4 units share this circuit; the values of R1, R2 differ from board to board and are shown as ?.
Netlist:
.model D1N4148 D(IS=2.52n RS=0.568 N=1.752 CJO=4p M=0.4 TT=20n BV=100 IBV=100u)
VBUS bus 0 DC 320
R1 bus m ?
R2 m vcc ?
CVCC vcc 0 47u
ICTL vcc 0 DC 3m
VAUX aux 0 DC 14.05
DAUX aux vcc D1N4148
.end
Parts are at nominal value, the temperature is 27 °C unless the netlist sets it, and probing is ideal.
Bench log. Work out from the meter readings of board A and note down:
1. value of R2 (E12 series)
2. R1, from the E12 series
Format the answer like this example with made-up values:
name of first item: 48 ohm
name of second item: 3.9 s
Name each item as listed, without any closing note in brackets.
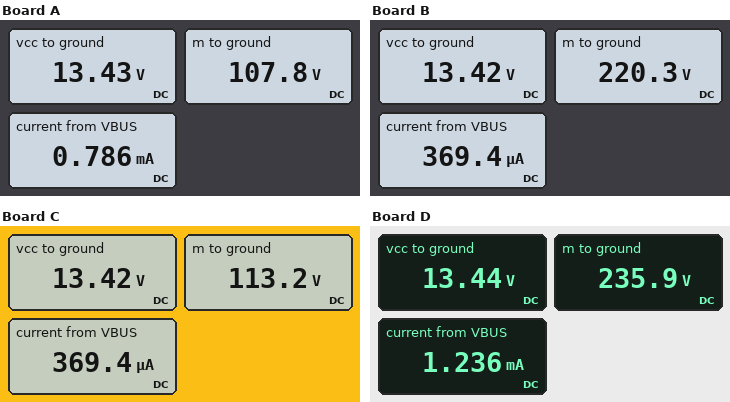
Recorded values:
value of R2: 120 kΩ
R1, from the E12 series: 270 kΩ
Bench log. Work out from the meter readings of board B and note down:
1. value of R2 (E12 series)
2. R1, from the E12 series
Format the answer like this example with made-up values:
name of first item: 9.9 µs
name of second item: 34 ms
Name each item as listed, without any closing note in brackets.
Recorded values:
value of R2: 560 kΩ
R1, from the E12 series: 270 kΩ
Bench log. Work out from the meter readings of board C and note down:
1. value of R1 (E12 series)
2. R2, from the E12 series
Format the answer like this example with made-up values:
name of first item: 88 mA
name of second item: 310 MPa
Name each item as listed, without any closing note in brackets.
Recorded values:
value of R1: 560 kΩ
R2, from the E12 series: 270 kΩ
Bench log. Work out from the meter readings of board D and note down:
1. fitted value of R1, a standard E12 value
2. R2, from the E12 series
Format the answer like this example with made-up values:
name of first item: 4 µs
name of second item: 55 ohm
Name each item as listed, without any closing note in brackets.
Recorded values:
fitted value of R1, a standard E12 value: 68 kΩ
R2, from the E12 series: 180 kΩ
